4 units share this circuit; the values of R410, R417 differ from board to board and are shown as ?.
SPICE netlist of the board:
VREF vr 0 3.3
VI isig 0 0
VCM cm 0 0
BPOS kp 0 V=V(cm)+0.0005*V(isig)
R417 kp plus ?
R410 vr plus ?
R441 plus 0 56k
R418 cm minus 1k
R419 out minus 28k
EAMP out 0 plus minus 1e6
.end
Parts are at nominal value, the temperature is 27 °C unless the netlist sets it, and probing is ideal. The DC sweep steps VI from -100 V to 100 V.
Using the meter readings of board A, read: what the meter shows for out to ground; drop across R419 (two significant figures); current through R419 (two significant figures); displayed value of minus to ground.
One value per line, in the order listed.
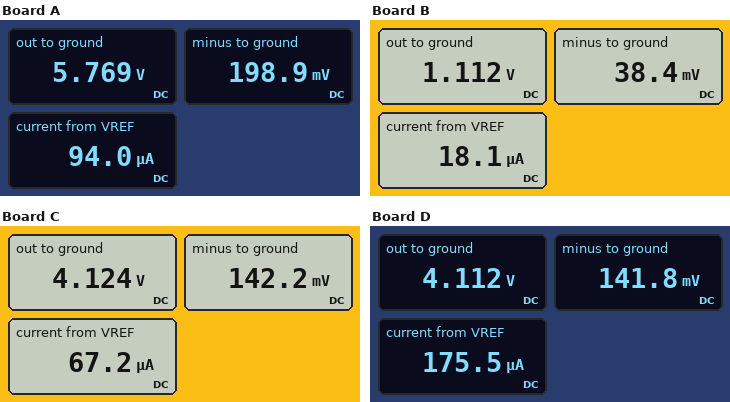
5.769 V
5.6 V
200 µA
198.9 mV
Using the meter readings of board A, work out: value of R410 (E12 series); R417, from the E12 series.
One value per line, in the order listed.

33 kΩ
2.2 kΩ
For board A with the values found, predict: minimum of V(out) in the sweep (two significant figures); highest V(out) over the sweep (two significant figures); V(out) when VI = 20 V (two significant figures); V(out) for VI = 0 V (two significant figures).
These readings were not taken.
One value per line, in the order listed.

4.5 V
7.1 V
6.0 V
5.8 V
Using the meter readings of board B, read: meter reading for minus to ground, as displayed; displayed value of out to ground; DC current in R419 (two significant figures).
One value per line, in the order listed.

38.4 mV
1.112 V
38 µA
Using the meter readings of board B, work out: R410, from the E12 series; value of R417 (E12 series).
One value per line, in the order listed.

180 kΩ
2.2 kΩ
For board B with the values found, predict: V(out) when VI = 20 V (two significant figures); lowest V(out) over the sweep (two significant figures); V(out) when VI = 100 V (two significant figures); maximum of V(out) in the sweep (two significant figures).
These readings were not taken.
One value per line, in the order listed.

1.4 V
-270 mV
2.5 V
2.5 V
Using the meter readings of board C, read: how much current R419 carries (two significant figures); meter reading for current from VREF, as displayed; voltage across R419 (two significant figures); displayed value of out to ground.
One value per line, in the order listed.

140 µA
67.2 µA
4.0 V
4.124 V
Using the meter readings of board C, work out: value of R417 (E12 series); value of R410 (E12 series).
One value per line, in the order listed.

2.2 kΩ
47 kΩ
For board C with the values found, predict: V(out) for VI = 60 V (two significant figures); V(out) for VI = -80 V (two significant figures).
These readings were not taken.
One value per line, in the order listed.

4.9 V
3.1 V
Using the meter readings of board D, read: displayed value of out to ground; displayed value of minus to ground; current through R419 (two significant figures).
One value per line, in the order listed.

4.112 V
141.8 mV
140 µA
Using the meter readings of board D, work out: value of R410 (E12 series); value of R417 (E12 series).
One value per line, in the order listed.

18 kΩ
820 Ω
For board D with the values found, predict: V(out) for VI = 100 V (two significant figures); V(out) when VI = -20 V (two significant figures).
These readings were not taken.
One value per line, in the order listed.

5.5 V
3.8 V
